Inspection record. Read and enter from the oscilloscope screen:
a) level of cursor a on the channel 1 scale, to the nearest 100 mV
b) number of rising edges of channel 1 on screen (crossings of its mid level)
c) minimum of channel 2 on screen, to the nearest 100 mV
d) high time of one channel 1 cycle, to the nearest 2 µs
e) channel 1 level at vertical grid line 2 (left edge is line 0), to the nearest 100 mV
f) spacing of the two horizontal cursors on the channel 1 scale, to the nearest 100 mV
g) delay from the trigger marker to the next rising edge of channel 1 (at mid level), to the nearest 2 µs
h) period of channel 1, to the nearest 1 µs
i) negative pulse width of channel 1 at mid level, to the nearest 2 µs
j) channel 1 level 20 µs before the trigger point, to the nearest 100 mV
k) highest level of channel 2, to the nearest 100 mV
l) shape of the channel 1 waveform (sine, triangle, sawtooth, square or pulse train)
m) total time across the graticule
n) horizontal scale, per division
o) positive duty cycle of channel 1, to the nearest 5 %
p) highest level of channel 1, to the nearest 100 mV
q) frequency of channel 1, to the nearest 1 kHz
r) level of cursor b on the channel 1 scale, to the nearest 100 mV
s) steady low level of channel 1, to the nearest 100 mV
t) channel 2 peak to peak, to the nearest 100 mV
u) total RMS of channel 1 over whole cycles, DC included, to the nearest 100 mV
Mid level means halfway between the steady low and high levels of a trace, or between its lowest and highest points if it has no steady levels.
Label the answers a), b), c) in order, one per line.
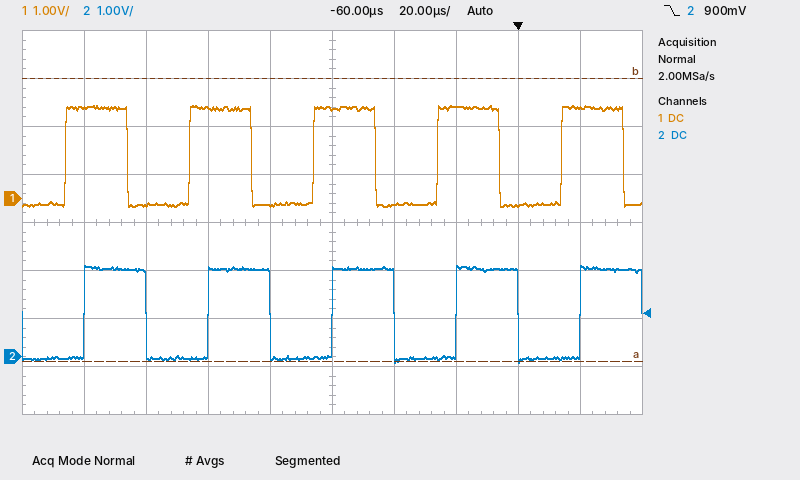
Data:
a) -3.4 V
b) 5
c) -100 mV
d) 20 µs
e) -100 mV
f) 5.9 V
g) 14 µs
h) 40 µs
i) 20 µs
j) 1.9 V
k) 1.9 V
l) square
m) 200 µs
n) 20 µs
o) 50 %
p) 1.9 V
q) 25 kHz
r) 2.5 V
s) -100 mV
t) 2.0 V
u) 1.3 V
